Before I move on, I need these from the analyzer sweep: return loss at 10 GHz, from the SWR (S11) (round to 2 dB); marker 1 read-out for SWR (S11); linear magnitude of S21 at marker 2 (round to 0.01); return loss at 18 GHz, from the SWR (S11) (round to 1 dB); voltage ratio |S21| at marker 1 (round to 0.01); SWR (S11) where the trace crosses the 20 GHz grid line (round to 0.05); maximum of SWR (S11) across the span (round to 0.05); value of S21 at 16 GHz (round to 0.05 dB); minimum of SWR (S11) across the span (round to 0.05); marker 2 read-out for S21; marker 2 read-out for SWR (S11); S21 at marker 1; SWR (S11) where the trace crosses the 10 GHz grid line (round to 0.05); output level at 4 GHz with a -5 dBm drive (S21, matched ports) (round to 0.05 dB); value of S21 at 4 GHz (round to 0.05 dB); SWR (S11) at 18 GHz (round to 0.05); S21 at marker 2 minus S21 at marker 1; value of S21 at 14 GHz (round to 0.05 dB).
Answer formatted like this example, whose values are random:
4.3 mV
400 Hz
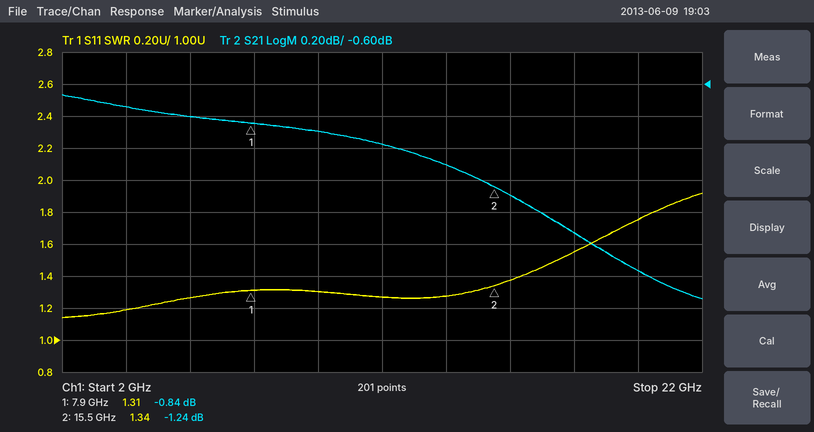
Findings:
18 dB
1.31
0.87
13 dB
0.91
1.75
1.90
-1.30 dB
1.15
-1.24 dB
1.34
-0.84 dB
1.30
-5.75 dBm
-0.75 dB
1.55
-0.40 dB
-1.10 dB
